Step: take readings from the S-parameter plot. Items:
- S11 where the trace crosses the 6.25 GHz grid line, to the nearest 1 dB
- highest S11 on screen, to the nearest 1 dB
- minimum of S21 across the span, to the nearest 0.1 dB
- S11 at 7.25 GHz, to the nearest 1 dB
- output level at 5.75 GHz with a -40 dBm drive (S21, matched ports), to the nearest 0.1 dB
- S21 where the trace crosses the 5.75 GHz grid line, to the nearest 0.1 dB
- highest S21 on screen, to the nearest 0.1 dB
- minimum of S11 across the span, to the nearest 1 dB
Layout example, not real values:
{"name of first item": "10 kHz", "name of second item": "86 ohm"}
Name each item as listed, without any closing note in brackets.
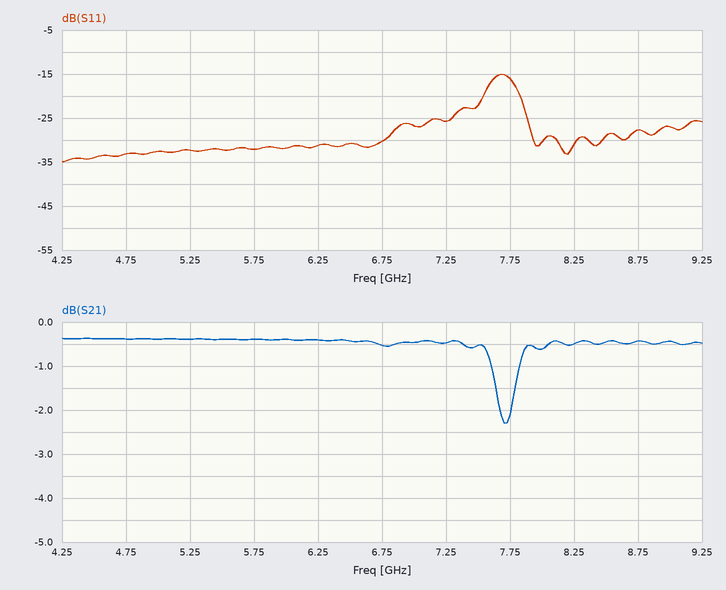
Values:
{"S11 where the trace crosses the 6.25 GHz grid line, to the nearest 1 dB": "-31 dB", "highest S11 on screen, to the nearest 1 dB": "-15 dB", "minimum of S21 across the span, to the nearest 0.1 dB": "-2.3 dB", "S11 at 7.25 GHz, to the nearest 1 dB": "-26 dB", "output level at 5.75 GHz with a -40 dBm drive (S21, matched ports), to the nearest 0.1 dB": "-40.4 dBm", "S21 where the trace crosses the 5.75 GHz grid line, to the nearest 0.1 dB": "-0.4 dB", "highest S21 on screen, to the nearest 0.1 dB": "-0.4 dB", "minimum of S11 across the span, to the nearest 1 dB": "-35 dB"}
